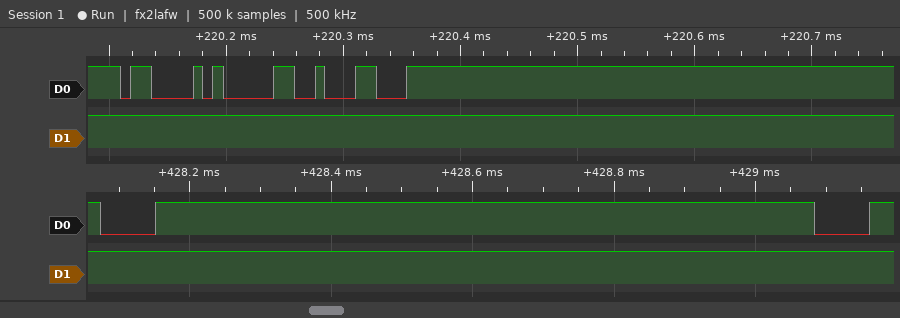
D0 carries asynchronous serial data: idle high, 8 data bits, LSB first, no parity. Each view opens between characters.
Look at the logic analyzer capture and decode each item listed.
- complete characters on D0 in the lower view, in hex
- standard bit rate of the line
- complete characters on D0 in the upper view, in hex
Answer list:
00, 00
115200 baud
43, 30, 8C
